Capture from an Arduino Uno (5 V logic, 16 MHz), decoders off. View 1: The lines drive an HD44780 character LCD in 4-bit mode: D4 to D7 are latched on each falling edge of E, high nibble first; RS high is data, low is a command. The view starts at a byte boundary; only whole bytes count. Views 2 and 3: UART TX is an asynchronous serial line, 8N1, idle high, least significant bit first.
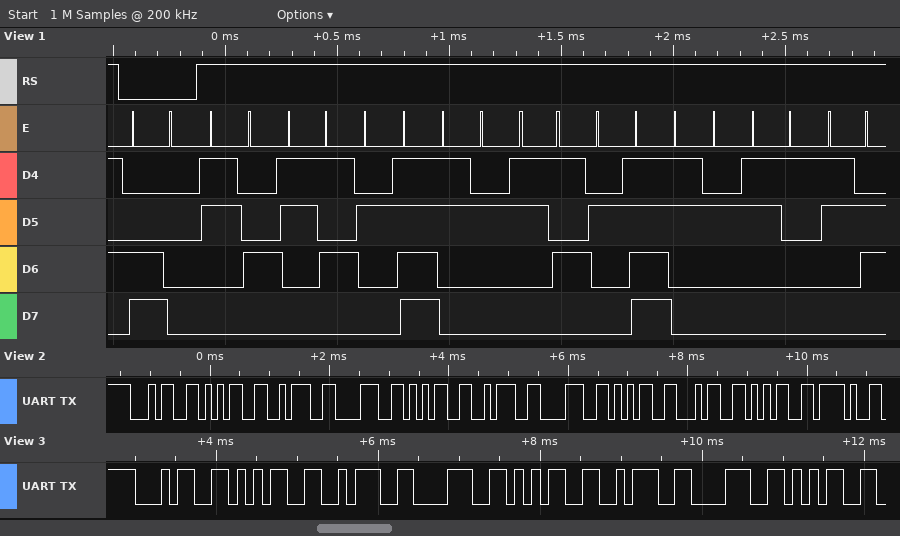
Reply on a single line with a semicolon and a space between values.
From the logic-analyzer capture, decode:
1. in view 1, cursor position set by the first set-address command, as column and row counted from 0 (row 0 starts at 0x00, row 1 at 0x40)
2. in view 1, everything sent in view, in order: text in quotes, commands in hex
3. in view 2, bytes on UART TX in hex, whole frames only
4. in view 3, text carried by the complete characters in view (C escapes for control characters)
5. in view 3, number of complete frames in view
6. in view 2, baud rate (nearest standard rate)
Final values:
column 0, row 1; 0xC0 "45/25/216"; 0x34 0x35 0x3A 0x38 0x35 0x3A 0x38 0x35 0x34 0x35 0x2F; "45:85:85"; 8; 9600 baud
